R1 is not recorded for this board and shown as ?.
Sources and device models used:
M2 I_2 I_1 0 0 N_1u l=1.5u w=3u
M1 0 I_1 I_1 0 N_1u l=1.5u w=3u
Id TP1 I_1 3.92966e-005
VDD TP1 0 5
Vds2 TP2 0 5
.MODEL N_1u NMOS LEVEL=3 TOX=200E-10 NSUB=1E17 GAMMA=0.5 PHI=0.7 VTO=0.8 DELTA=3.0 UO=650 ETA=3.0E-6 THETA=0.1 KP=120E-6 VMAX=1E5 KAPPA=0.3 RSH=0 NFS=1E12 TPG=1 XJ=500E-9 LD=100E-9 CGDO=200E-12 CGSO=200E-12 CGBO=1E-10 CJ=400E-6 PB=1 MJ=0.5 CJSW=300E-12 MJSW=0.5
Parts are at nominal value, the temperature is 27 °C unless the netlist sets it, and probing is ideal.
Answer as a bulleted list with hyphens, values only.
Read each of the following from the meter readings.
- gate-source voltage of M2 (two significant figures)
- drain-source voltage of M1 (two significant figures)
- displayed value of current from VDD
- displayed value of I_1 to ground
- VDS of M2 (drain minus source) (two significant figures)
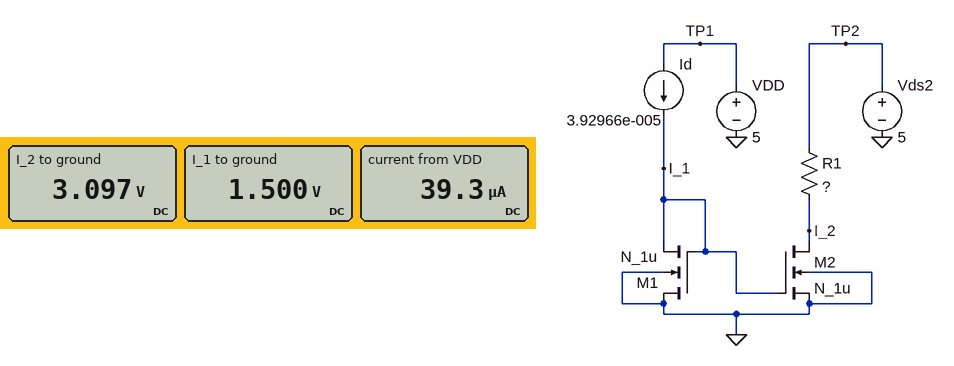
- 1.5 V
- -1.5 V
- 39.3 µA
- 1.500 V
- 3.1 V
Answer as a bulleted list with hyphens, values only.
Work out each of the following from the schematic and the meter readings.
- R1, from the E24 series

- 47 kΩ
